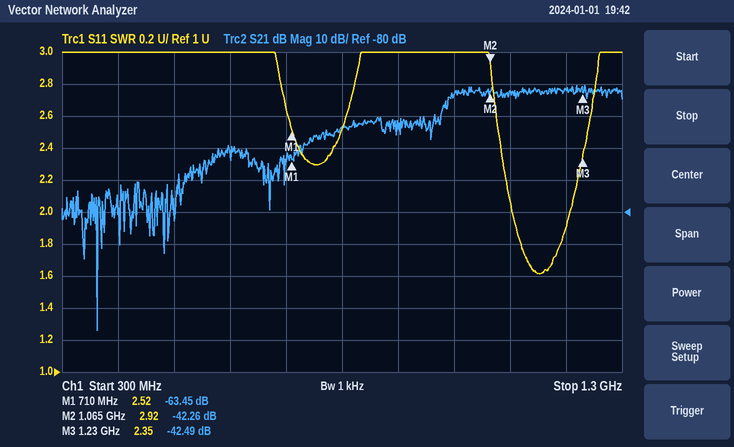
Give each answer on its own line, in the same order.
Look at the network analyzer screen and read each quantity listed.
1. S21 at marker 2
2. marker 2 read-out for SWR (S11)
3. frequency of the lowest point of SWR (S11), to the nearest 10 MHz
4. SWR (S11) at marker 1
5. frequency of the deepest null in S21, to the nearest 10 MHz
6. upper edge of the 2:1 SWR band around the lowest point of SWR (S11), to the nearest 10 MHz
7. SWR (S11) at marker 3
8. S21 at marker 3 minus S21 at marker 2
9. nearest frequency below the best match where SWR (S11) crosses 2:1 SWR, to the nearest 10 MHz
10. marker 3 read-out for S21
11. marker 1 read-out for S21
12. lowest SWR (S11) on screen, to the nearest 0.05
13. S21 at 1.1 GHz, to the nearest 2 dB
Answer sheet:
-42.26 dB
2.92
1.15 GHz
2.52
360 MHz
1.21 GHz
2.35
-0.23 dB
1.10 GHz
-42.49 dB
-63.45 dB
1.60
-42 dB
